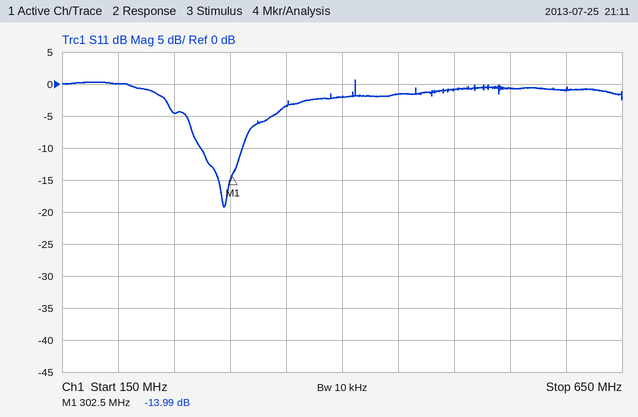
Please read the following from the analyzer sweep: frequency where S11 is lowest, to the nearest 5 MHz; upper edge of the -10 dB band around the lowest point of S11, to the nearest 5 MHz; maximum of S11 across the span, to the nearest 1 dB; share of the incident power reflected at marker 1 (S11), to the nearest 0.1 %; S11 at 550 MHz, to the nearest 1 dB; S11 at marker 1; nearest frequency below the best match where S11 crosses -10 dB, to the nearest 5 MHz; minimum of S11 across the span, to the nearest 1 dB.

295 MHz
310 MHz
1 dB
4.0 %
-1 dB
-13.99 dB
275 MHz
-19 dB
